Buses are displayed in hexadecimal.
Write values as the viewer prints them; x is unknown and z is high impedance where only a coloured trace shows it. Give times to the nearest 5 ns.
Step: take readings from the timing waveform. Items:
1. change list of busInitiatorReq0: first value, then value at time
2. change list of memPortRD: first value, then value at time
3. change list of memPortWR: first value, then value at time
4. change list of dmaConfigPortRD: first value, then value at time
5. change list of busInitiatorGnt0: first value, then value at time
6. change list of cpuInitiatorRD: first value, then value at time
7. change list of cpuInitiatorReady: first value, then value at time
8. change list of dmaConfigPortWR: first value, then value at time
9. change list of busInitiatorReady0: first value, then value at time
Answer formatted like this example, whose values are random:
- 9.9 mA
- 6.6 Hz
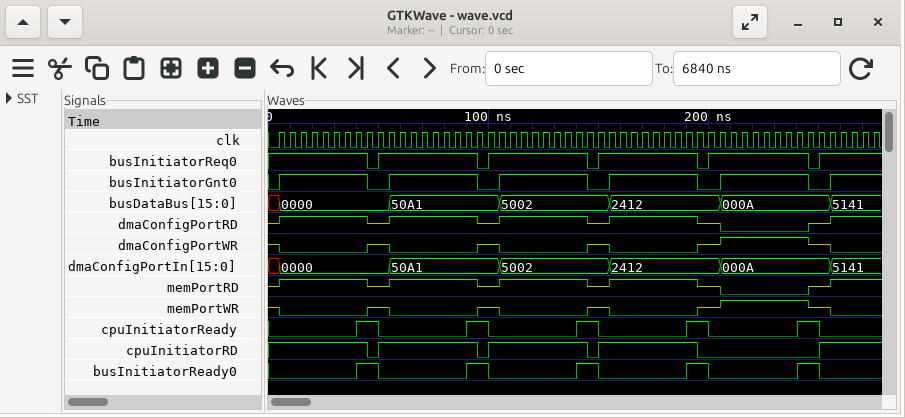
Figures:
- 1, 0 at 45 ns, 1 at 50 ns, 0 at 95 ns, 1 at 100 ns, 0 at 145 ns, 1 at 150 ns, 0 at 195 ns, 1 at 200 ns, 0 at 245 ns, 1 at 250 ns
- z, 1 at 5 ns, z at 45 ns, 1 at 55 ns, z at 95 ns, 1 at 105 ns, z at 145 ns, 1 at 155 ns, z at 195 ns, 0 at 205 ns, z at 245 ns, 1 at 255 ns
- z, 0 at 5 ns, z at 45 ns, 0 at 55 ns, z at 95 ns, 0 at 105 ns, z at 145 ns, 0 at 155 ns, z at 195 ns, 1 at 205 ns, z at 245 ns, 0 at 255 ns
- z, 1 at 5 ns, z at 45 ns, 1 at 55 ns, z at 95 ns, 1 at 105 ns, z at 145 ns, 1 at 155 ns, z at 195 ns, 0 at 205 ns, z at 245 ns, 1 at 255 ns
- 0, 1 at 5 ns, 0 at 45 ns, 1 at 55 ns, 0 at 95 ns, 1 at 105 ns, 0 at 145 ns, 1 at 155 ns, 0 at 195 ns, 1 at 205 ns, 0 at 245 ns, 1 at 255 ns
- 1, 0 at 45 ns, 1 at 50 ns, 0 at 95 ns, 1 at 100 ns, 0 at 145 ns, 1 at 150 ns, 0 at 195 ns, 1 at 250 ns
- 0, 1 at 40 ns, 0 at 50 ns, 1 at 90 ns, 0 at 100 ns, 1 at 140 ns, 0 at 150 ns, 1 at 190 ns, 0 at 200 ns, 1 at 240 ns, 0 at 250 ns
- z, 0 at 5 ns, z at 45 ns, 0 at 55 ns, z at 95 ns, 0 at 105 ns, z at 145 ns, 0 at 155 ns, z at 195 ns, 1 at 205 ns, z at 245 ns, 0 at 255 ns
- 0, 1 at 40 ns, 0 at 50 ns, 1 at 90 ns, 0 at 100 ns, 1 at 140 ns, 0 at 150 ns, 1 at 190 ns, 0 at 200 ns, 1 at 240 ns, 0 at 250 ns
